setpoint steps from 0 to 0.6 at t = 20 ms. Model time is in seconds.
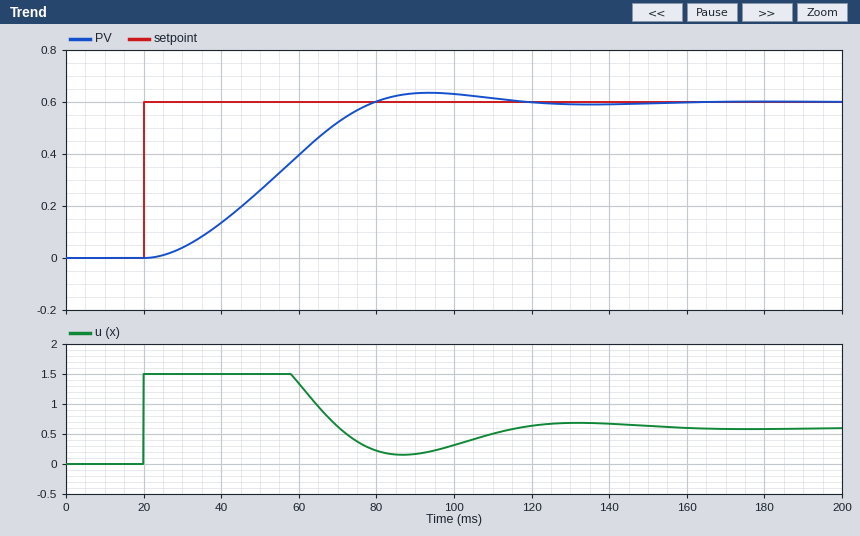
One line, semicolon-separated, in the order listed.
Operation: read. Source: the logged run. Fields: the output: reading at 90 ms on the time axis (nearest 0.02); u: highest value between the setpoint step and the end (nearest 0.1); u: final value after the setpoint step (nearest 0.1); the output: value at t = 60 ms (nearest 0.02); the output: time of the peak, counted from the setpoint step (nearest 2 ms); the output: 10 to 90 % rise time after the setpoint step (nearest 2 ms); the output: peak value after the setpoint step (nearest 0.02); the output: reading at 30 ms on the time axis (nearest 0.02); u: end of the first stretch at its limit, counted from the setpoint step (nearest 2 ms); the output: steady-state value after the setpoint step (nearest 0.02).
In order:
0.64; 1.5; 0.6; 0.40; 74 ms; 40 ms; 0.64; 0.04; 38 ms; 0.60
